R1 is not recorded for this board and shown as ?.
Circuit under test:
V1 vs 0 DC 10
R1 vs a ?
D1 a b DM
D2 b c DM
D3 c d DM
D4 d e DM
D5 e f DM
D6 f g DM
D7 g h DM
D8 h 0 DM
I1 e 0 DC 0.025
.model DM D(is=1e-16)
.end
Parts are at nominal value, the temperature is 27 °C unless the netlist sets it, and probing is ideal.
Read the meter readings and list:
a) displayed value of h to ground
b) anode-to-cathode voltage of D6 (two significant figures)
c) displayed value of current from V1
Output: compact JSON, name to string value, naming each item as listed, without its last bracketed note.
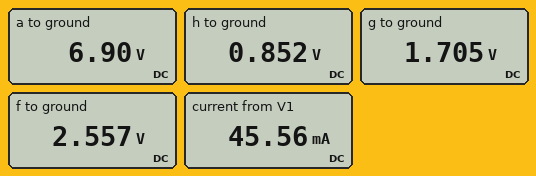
{"displayed value of h to ground": "0.852 V", "anode-to-cathode voltage of D6": "850 mV", "displayed value of current from V1": "45.56 mA"}
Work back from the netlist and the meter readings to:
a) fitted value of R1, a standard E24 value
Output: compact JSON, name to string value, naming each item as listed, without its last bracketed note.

{"fitted value of R1, a standard E24 value": "68 Ω"}
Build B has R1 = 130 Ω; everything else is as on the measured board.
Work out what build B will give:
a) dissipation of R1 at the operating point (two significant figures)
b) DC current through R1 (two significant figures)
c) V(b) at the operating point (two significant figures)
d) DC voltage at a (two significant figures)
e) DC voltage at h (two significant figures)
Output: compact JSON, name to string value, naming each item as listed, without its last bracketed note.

{"dissipation of R1 at the operating point": "91 mW", "DC current through R1": "26 mA", "V(b) at the operating point": "5.7 V", "DC voltage at a": "6.6 V", "DC voltage at h": "780 mV"}
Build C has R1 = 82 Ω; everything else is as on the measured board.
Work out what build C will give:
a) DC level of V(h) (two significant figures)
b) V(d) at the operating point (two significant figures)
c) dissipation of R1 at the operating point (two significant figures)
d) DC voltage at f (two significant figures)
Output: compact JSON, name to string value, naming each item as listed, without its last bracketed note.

{"DC level of V(h)": "840 mV", "V(d) at the operating point": "4.2 V", "dissipation of R1 at the operating point": "120 mW", "DC voltage at f": "2.5 V"}
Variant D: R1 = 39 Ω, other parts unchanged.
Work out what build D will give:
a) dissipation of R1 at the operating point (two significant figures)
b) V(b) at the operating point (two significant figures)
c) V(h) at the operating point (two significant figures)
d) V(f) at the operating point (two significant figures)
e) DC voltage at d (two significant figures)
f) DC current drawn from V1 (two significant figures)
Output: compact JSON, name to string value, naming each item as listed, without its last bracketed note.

{"dissipation of R1 at the operating point": "220 mW", "V(b) at the operating point": "6.2 V", "V(h) at the operating point": "880 mV", "V(f) at the operating point": "2.6 V", "DC voltage at d": "4.4 V", "DC current drawn from V1": "76 mA"}
